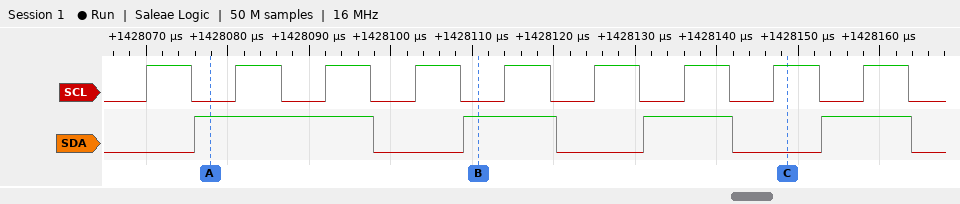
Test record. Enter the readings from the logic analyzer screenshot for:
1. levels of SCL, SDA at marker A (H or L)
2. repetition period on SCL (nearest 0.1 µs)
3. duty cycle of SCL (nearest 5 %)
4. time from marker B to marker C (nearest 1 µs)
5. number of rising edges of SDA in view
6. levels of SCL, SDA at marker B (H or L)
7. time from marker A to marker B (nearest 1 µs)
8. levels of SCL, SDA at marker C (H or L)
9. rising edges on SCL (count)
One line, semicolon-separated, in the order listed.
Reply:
SCL=L, SDA=H; 11 µs; 50 %; 38 µs; 4; SCL=L, SDA=H; 33 µs; SCL=H, SDA=L; 9
